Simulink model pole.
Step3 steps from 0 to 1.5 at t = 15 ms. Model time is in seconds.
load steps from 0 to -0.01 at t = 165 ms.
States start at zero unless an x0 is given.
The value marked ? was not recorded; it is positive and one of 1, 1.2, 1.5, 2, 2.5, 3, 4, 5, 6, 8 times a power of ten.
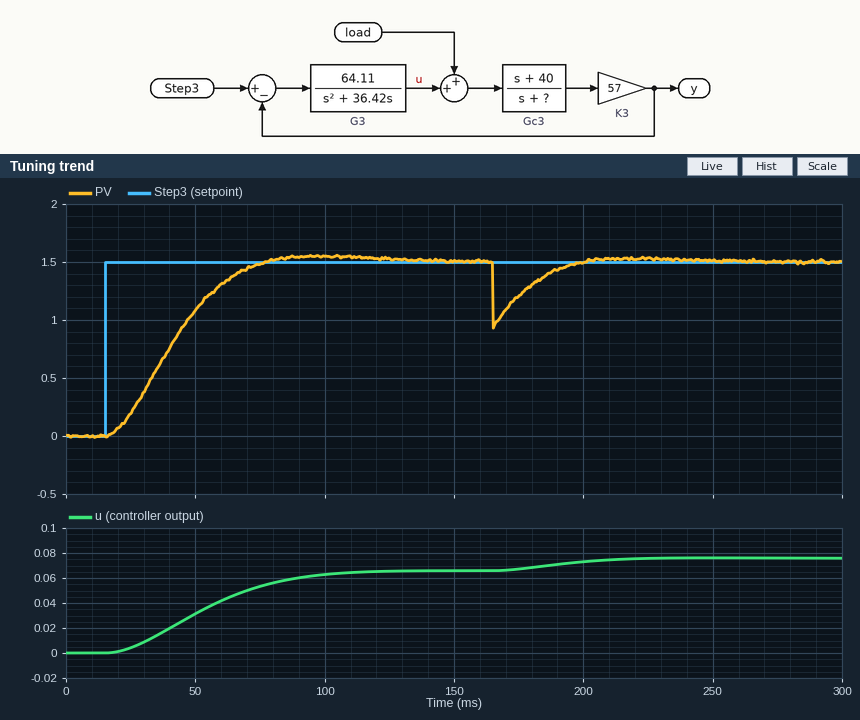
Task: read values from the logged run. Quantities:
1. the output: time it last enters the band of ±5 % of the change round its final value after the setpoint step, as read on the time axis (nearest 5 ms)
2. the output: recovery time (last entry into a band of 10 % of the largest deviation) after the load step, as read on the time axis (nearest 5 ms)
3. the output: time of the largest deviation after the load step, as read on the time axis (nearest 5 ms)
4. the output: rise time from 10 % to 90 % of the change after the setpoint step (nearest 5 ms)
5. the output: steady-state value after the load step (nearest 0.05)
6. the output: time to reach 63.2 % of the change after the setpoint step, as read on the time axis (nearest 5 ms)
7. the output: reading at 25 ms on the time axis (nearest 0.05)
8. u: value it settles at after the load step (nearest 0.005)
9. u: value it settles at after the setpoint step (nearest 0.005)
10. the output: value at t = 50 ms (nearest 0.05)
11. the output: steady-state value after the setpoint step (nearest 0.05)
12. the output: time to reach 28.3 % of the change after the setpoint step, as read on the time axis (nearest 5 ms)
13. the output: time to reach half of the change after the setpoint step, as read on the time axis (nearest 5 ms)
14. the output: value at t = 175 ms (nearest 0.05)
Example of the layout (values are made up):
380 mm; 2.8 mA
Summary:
70 ms; 190 ms; 165 ms; 40 ms; 1.50; 45 ms; 0.20; 0.075; 0.065; 1.10; 1.50; 30 ms; 40 ms; 1.20
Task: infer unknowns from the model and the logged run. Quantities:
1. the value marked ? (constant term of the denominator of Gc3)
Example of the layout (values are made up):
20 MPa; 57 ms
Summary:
100
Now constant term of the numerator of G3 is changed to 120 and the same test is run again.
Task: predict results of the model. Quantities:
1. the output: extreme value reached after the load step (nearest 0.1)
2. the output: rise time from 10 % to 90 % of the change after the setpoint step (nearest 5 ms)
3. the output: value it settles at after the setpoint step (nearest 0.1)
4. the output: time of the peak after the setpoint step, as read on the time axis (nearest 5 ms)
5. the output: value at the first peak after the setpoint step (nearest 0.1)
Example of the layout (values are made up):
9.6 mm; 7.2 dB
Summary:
0.9; 20 ms; 1.5; 60 ms; 1.7
